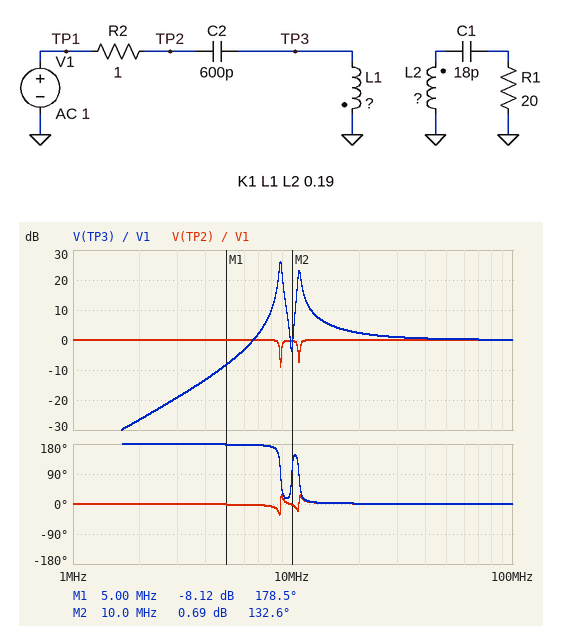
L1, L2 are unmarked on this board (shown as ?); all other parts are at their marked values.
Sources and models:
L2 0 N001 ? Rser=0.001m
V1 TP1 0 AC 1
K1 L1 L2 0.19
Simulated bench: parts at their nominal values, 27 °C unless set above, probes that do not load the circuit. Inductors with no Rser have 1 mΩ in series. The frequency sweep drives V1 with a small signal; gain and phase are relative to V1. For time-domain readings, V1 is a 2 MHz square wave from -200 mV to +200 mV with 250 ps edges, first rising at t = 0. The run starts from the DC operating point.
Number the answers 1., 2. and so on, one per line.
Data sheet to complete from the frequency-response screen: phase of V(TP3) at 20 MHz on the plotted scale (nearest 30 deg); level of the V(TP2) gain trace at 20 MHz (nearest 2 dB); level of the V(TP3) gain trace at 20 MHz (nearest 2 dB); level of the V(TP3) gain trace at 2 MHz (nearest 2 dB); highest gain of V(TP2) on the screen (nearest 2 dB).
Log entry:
1. 0 deg
2. 0 dB
3. 2 dB
4. -26 dB
5. 0 dB
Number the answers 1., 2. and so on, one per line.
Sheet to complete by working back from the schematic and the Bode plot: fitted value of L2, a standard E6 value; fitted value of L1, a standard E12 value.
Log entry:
1. 15 µH
2. 470 nH
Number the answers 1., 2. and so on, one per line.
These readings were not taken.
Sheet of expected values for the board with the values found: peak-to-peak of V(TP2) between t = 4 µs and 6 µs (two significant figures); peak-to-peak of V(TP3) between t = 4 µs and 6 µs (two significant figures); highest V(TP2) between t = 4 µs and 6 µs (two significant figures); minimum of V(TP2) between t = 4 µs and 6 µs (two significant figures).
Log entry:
1. 410 mV
2. 510 mV
3. 210 mV
4. -210 mV
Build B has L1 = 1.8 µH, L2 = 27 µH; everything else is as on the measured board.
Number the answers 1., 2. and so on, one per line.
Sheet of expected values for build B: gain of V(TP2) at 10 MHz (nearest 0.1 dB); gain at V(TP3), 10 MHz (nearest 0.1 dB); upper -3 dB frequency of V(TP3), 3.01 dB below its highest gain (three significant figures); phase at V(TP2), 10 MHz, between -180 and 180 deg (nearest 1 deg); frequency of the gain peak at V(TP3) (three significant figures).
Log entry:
1. 0 dB
2. 2.5 dB
3. 4.82 MHz
4. 1 deg
5. 4.78 MHz
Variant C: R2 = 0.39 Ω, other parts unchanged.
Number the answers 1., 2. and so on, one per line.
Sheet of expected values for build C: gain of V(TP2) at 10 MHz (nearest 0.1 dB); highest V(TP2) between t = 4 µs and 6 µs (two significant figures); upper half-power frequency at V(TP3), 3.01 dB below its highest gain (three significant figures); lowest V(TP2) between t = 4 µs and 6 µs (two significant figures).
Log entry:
1. -0.1 dB
2. 200 mV
3. 8.85 MHz
4. -200 mV
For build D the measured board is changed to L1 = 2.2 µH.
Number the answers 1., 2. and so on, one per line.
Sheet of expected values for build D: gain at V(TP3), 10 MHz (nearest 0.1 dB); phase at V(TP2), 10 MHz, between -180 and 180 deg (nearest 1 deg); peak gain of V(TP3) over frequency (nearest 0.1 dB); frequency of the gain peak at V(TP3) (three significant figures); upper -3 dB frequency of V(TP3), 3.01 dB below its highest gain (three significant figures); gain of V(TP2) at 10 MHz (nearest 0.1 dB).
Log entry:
1. 3.5 dB
2. 1 deg
3. 35.6 dB
4. 4.36 MHz
5. 4.40 MHz
6. -0.1 dB
